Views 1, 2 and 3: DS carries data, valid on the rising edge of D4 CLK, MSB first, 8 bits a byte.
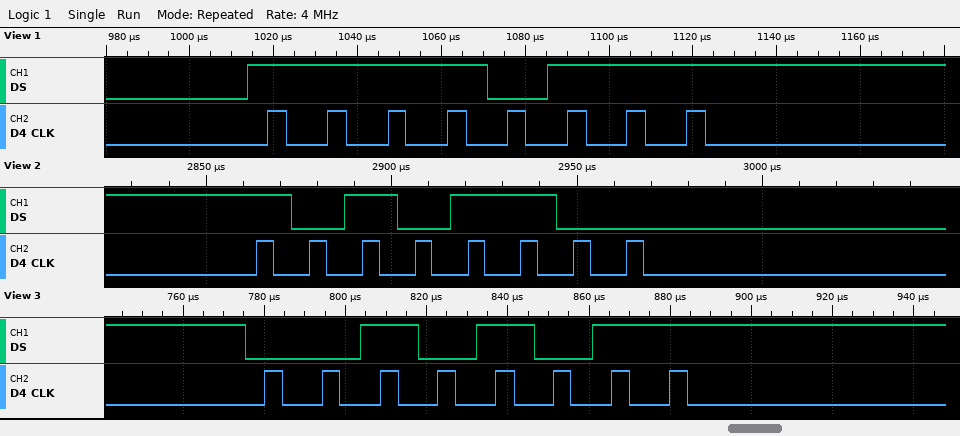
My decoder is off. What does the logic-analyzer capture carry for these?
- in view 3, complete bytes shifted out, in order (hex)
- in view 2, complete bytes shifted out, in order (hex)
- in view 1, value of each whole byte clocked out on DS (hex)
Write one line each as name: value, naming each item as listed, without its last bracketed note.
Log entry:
in view 3, complete bytes shifted out, in order: 2B
in view 2, complete bytes shifted out, in order: AC
in view 1, value of each whole byte clocked out on DS: 0xF7
